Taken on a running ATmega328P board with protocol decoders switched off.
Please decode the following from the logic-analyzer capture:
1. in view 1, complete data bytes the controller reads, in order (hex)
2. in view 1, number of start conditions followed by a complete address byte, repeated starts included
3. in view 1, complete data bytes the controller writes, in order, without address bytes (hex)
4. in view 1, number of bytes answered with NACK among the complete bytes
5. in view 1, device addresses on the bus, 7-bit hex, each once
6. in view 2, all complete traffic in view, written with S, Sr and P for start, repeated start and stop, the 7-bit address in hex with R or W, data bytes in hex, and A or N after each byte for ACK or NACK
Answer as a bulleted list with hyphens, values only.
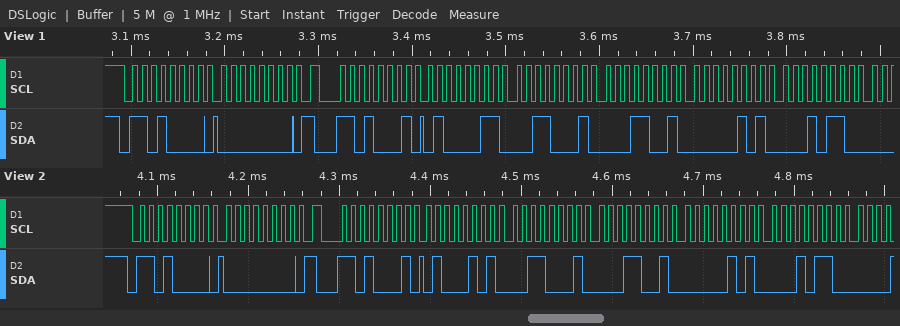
- 43 31 19 05 16
- 2
- 00
- 0
- 0x68
- S 68W A 00 A Sr 68R A 45 A 31 A 19 A 05 A 16 A
